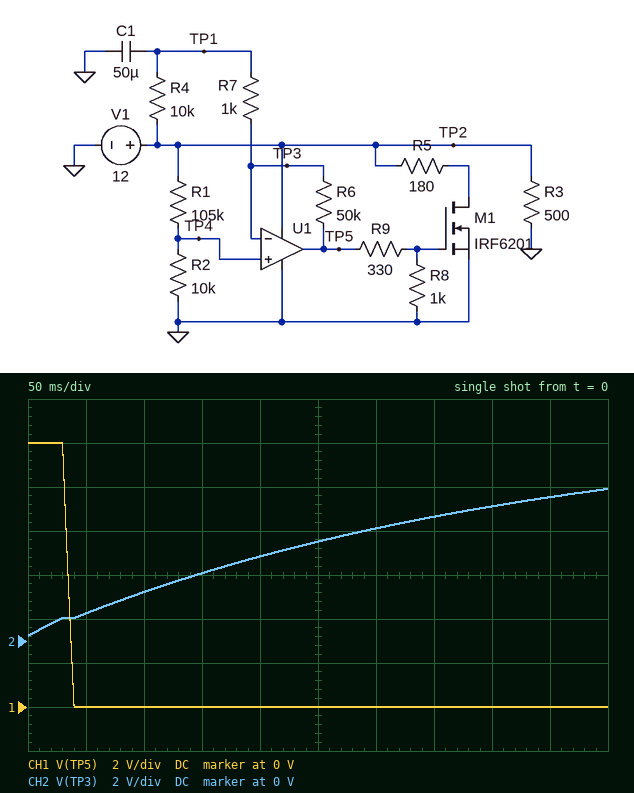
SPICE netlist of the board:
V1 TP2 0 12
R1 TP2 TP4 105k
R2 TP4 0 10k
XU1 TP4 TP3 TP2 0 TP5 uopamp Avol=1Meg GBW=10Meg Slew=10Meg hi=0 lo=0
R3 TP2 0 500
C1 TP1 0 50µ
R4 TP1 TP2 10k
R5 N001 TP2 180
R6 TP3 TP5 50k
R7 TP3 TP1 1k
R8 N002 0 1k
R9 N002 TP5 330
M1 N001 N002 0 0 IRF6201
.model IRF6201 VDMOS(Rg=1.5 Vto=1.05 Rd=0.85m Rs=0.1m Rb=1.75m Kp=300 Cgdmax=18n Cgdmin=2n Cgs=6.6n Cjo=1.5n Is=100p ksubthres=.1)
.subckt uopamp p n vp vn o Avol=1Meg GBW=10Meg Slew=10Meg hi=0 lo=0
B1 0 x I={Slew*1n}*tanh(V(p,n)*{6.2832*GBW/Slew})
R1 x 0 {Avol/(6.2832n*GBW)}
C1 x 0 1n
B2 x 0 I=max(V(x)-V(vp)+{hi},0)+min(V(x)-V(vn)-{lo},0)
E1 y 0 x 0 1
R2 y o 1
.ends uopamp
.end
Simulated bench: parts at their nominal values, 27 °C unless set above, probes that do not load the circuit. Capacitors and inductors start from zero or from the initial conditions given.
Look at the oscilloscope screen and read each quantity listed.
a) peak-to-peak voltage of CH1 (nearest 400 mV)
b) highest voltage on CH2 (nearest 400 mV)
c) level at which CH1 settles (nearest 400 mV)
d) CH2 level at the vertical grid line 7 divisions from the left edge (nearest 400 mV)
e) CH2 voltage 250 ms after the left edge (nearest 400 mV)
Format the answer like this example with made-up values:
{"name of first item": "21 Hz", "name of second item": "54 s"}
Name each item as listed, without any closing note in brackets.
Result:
{"peak-to-peak voltage of CH1": "12.0 V", "highest voltage on CH2": "6.8 V", "level at which CH1 settles": "0 V", "CH2 level at the vertical grid line 7 divisions from the left edge": "5.6 V", "CH2 voltage 250 ms after the left edge": "4.4 V"}
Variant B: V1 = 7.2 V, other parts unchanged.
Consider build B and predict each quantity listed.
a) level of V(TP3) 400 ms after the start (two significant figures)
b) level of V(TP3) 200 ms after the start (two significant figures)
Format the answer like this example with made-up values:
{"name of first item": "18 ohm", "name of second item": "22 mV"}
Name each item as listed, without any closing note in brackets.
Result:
{"level of V(TP3) 400 ms after the start": "3.7 V", "level of V(TP3) 200 ms after the start": "2.3 V"}
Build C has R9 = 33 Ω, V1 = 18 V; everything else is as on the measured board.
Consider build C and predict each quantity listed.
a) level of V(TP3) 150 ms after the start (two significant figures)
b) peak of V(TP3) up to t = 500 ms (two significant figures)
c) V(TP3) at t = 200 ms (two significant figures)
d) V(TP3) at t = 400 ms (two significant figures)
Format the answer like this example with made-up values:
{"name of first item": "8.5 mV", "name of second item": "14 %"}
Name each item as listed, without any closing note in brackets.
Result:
{"level of V(TP3) 150 ms after the start": "4.6 V", "peak of V(TP3) up to t = 500 ms": "10 V", "V(TP3) at t = 200 ms": "5.8 V", "V(TP3) at t = 400 ms": "9.2 V"}
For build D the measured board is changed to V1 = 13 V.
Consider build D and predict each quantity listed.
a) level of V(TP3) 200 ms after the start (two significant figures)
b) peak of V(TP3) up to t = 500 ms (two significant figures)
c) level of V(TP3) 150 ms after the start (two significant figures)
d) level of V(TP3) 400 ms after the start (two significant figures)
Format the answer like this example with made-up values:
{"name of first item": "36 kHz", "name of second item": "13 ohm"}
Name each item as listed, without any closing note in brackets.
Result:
{"level of V(TP3) 200 ms after the start": "4.2 V", "peak of V(TP3) up to t = 500 ms": "7.5 V", "level of V(TP3) 150 ms after the start": "3.3 V", "level of V(TP3) 400 ms after the start": "6.6 V"}
